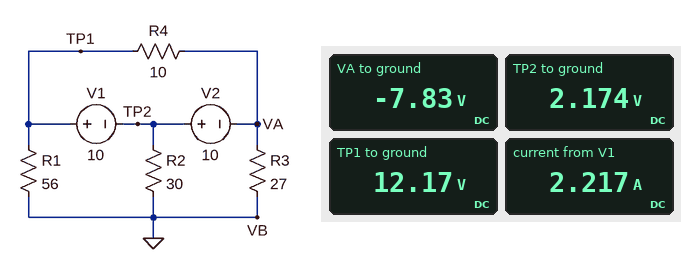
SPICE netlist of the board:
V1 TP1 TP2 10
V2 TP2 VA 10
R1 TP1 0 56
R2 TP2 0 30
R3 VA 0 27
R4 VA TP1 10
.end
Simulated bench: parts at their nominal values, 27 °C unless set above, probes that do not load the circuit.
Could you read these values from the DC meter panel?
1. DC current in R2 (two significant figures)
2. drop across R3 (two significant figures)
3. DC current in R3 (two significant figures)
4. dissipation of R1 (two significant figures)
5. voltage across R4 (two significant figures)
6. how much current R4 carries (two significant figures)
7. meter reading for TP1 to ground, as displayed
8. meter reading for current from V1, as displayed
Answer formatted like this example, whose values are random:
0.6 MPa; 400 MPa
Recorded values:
72 mA; 7.8 V; 290 mA; 2.6 W; 20 V; 2.0 A; 12.17 V; 2.217 A
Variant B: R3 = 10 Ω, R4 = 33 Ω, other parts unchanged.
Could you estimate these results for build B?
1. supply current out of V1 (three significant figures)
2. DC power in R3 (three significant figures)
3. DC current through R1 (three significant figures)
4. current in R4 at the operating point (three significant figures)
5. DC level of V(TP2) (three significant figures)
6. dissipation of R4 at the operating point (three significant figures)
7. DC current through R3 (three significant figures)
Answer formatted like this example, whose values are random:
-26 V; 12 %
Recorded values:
882 mA; 2.09 W; 276 mA; 606 mA; 5.43 V; 12.1 W; 457 mA
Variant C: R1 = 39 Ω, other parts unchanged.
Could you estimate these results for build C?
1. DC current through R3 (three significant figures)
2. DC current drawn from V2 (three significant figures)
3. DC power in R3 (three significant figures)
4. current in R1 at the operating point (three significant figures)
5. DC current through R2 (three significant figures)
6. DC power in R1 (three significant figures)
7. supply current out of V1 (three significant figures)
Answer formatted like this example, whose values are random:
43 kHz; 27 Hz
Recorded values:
326 mA; 2.33 A; 2.88 W; 287 mA; 39.6 mA; 3.21 W; 2.29 A
